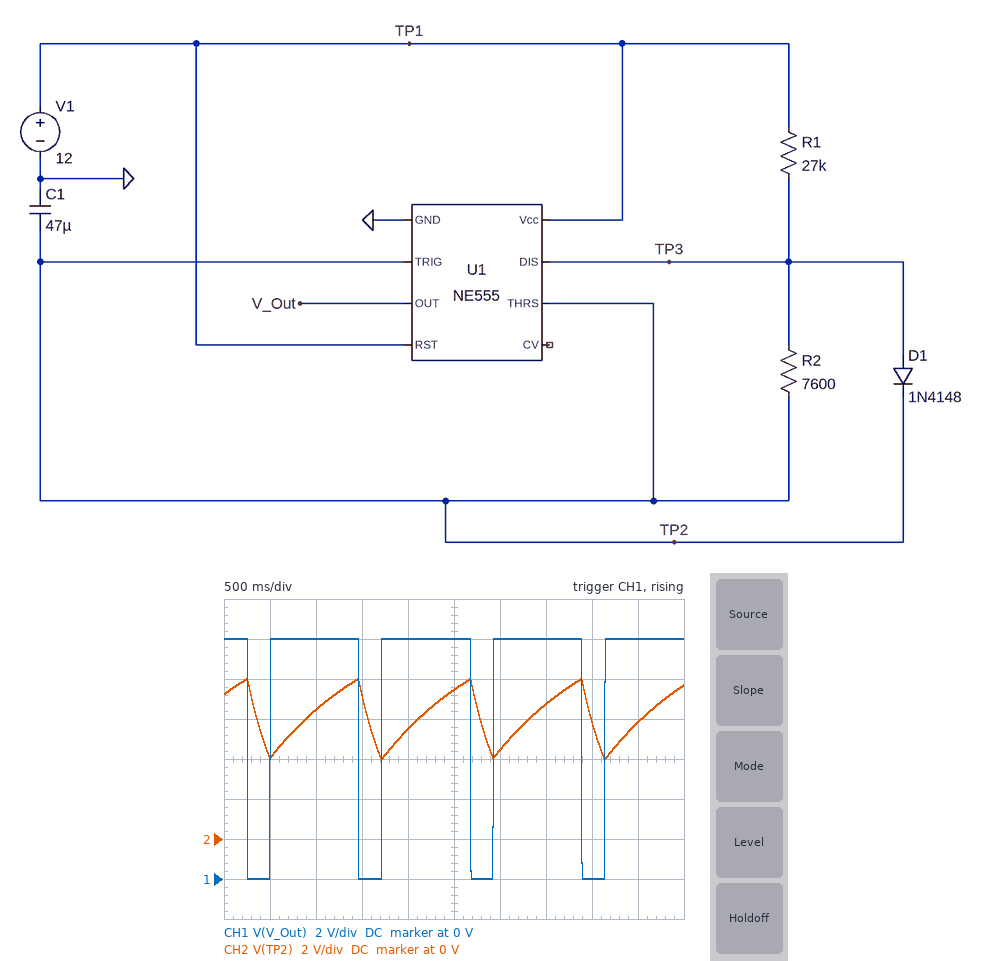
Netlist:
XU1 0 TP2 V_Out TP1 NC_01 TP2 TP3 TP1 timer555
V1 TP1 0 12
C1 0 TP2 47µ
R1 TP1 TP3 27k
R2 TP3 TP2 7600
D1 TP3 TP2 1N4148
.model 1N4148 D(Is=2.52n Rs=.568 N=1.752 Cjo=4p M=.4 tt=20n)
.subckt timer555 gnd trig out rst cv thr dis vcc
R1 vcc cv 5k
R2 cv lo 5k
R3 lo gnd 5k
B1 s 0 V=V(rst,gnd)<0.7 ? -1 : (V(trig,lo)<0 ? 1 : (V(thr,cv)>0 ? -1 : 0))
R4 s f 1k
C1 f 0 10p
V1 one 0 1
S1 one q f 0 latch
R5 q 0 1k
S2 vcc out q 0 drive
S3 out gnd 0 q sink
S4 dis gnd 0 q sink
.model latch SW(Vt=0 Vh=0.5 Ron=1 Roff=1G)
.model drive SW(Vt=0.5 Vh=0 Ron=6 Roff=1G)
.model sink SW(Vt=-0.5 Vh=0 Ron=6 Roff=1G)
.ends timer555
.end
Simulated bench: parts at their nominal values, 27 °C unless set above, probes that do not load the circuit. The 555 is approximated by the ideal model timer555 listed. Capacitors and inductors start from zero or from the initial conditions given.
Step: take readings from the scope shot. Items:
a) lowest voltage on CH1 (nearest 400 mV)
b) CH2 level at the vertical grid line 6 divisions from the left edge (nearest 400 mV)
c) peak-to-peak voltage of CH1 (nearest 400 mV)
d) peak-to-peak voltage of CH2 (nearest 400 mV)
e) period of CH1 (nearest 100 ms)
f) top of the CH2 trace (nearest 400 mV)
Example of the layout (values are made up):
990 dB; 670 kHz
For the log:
0 V; 4.4 V; 12.0 V; 4.0 V; 1.2 s; 8.0 V
